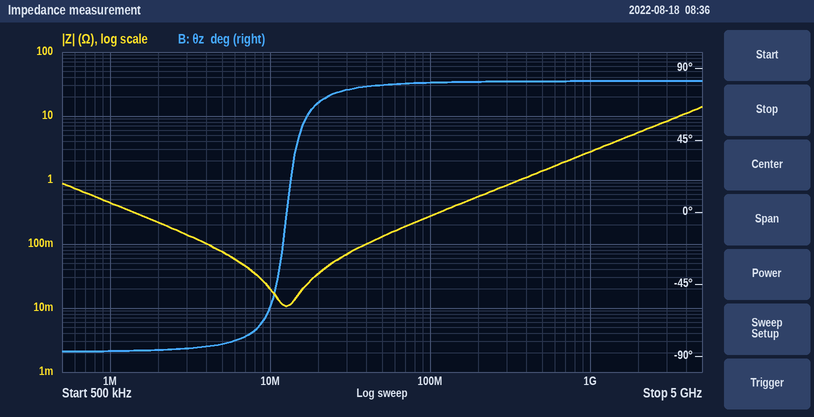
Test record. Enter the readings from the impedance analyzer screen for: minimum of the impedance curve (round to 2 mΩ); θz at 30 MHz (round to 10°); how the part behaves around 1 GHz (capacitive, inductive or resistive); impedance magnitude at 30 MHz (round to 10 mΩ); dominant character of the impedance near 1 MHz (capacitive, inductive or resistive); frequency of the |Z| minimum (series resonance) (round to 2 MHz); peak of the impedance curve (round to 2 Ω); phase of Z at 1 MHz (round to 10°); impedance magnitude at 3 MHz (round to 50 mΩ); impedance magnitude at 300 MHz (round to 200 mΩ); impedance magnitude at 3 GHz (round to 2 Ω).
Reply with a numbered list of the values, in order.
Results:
1. 10 mΩ
2. 80°
3. inductive
4. 70 mΩ
5. capacitive
6. 12 MHz
7. 14 Ω
8. -90°
9. 150 mΩ
10. 800 mΩ
11. 8 Ω
